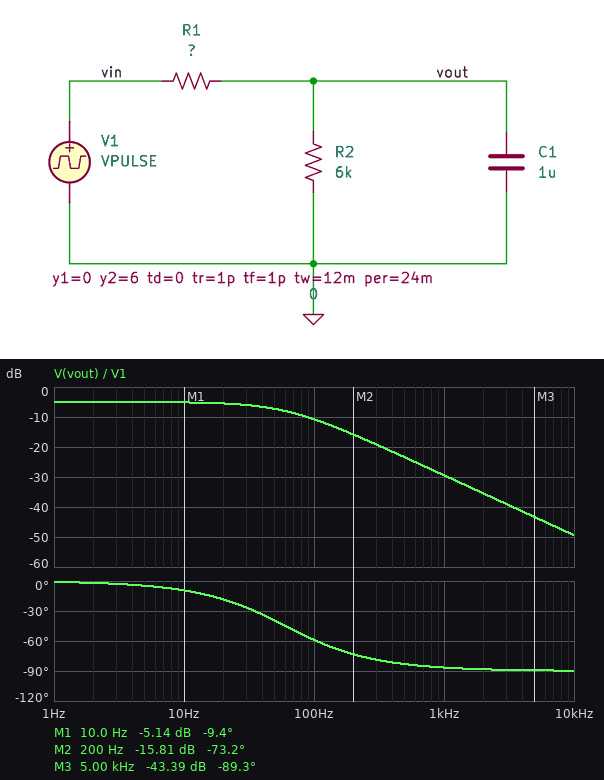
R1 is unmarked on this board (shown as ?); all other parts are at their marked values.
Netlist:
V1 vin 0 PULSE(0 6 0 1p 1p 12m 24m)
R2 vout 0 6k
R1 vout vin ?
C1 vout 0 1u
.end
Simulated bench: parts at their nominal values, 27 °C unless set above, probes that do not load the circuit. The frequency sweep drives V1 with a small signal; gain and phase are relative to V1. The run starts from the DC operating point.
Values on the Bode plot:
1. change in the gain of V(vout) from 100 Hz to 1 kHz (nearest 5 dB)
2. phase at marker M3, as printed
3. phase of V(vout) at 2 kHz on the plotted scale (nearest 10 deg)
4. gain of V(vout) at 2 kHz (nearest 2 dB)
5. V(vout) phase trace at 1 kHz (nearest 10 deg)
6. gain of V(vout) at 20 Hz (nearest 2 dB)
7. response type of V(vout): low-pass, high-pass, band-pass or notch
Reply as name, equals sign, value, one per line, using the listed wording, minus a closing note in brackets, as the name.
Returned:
change in the gain of V(vout) from 100 Hz to 1 kHz = -20 dB
phase at marker M3, as printed = -89.3 deg
phase of V(vout) at 2 kHz on the plotted scale = -90 deg
gain of V(vout) at 2 kHz = -36 dB
V(vout) phase trace at 1 kHz = -90 deg
gain of V(vout) at 20 Hz = -6 dB
response type of V(vout): low-pass, high-pass, band-pass or notch = low-pass
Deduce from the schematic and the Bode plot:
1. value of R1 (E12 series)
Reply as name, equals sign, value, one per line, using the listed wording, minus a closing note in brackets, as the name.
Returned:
value of R1 = 4.7 kΩ
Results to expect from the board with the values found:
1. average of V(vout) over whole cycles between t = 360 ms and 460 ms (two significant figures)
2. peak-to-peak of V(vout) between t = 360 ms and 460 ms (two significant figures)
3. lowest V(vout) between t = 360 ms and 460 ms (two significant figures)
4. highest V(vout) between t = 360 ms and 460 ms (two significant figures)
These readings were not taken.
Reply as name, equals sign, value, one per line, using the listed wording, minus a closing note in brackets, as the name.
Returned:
average of V(vout) over whole cycles between t = 360 ms and 460 ms = 1.7 V
peak-to-peak of V(vout) between t = 360 ms and 460 ms = 3.3 V
lowest V(vout) between t = 360 ms and 460 ms = 35 mV
highest V(vout) between t = 360 ms and 460 ms = 3.3 V
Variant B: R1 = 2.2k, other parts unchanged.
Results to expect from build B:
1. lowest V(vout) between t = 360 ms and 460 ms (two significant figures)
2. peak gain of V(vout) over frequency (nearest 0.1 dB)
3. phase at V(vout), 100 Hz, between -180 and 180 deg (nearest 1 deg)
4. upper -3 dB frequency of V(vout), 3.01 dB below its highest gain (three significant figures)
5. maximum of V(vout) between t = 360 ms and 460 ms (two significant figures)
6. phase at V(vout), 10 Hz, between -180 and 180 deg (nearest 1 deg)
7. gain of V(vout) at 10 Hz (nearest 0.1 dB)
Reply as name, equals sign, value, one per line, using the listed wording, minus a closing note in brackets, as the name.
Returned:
lowest V(vout) between t = 360 ms and 460 ms = 2.5 mV
peak gain of V(vout) over frequency = -2.7 dB
phase at V(vout), 100 Hz, between -180 and 180 deg = -45 deg
upper -3 dB frequency of V(vout), 3.01 dB below its highest gain = 98.9 Hz
maximum of V(vout) between t = 360 ms and 460 ms = 4.4 V
phase at V(vout), 10 Hz, between -180 and 180 deg = -6 deg
gain of V(vout) at 10 Hz = -2.8 dB
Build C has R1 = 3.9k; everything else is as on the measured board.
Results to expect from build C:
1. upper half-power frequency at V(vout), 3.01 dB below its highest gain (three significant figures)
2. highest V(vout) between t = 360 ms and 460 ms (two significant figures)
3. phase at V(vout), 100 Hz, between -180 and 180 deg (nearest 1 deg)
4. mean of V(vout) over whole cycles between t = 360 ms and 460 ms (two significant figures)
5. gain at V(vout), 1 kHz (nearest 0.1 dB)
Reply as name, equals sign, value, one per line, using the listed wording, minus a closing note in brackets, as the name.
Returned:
upper half-power frequency at V(vout), 3.01 dB below its highest gain = 67.3 Hz
highest V(vout) between t = 360 ms and 460 ms = 3.6 V
phase at V(vout), 100 Hz, between -180 and 180 deg = -56 deg
mean of V(vout) over whole cycles between t = 360 ms and 460 ms = 1.8 V
gain at V(vout), 1 kHz = -27.8 dB
